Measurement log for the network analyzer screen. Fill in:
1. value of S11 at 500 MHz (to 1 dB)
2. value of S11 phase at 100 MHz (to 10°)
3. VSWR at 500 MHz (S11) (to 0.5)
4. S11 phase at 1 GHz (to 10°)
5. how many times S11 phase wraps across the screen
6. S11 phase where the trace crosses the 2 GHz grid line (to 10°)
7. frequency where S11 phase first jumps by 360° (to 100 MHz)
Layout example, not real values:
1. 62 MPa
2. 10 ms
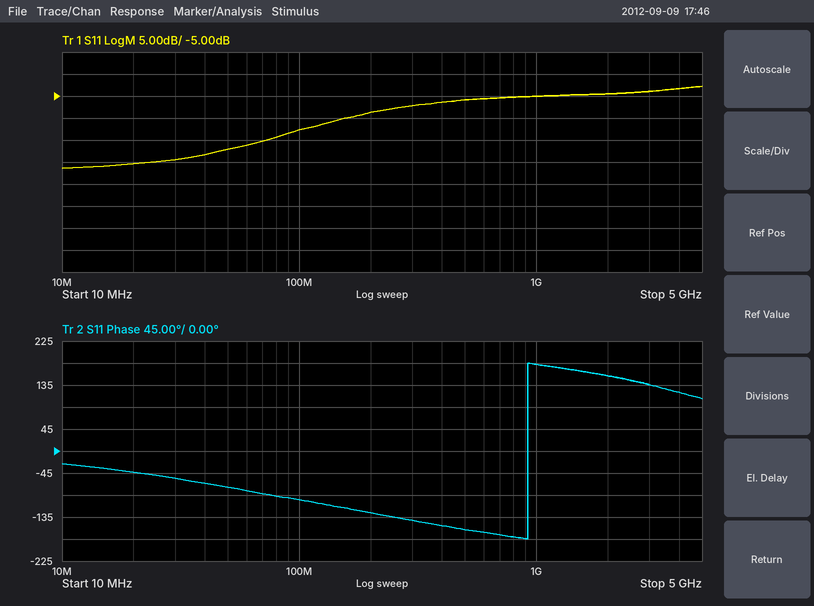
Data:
1. -6 dB
2. -100°
3. 3.0
4. 180°
5. 1
6. 150°
7. 900 MHz
